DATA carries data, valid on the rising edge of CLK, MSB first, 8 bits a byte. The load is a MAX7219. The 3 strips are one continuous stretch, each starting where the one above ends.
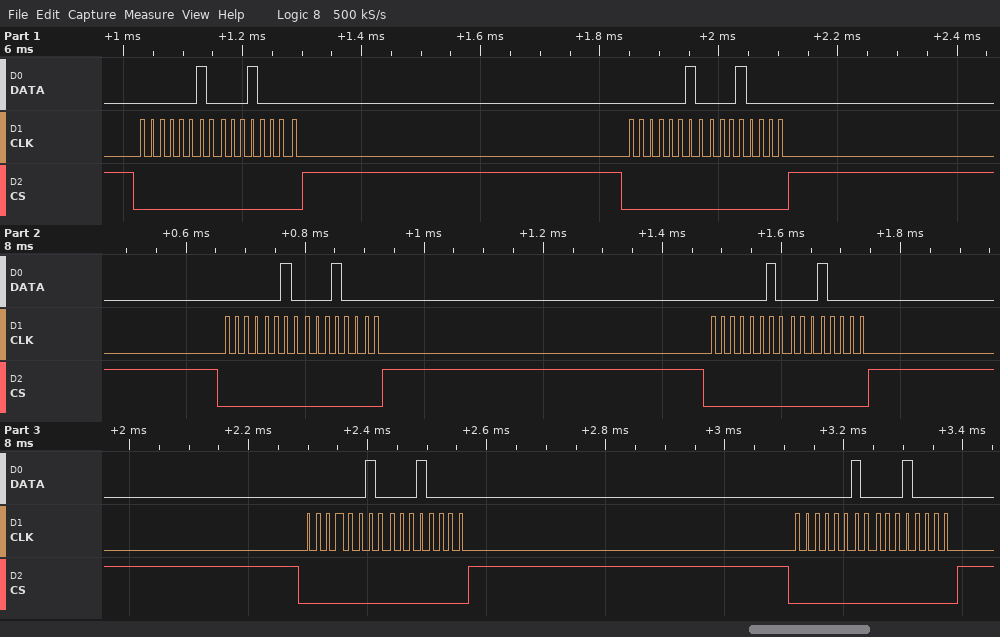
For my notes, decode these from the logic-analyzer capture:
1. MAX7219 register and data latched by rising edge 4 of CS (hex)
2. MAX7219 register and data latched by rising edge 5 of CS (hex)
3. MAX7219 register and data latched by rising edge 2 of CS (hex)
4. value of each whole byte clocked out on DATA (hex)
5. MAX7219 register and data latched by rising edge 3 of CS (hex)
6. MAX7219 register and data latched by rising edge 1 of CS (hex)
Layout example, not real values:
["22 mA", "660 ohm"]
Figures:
["register 0x2, data 0x10", "register 0x2, data 0x10", "register 0x2, data 0x10", "02 10 02 10 02 10 02 10 02 10 02 10", "register 0x2, data 0x10", "register 0x2, data 0x10"]
